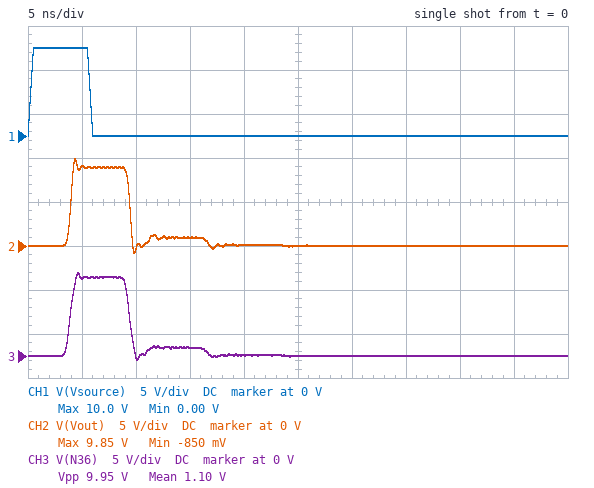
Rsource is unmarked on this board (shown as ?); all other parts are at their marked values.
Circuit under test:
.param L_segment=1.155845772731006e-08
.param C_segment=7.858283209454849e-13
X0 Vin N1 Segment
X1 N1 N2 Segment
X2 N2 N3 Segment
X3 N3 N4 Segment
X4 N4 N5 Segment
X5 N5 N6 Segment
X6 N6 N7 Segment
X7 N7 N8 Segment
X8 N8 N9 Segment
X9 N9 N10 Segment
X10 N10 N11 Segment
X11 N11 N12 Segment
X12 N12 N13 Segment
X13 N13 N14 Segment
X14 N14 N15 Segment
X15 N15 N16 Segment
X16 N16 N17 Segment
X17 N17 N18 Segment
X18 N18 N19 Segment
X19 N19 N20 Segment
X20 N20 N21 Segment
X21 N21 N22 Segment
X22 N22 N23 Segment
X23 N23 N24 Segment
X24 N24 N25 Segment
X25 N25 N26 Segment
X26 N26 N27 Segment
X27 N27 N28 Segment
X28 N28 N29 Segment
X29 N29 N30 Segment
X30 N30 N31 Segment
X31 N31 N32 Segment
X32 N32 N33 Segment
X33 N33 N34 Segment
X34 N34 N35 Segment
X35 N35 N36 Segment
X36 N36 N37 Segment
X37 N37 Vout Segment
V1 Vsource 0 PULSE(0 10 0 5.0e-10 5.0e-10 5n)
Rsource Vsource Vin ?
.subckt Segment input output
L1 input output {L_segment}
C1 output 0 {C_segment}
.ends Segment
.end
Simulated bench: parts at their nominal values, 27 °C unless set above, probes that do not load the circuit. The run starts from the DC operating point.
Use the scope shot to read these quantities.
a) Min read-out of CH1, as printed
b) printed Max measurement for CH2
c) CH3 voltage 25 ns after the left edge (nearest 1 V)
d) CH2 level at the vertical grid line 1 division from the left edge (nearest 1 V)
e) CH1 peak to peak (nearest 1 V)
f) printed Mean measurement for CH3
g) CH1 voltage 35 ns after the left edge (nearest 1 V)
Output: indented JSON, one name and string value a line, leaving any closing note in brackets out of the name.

{
  "Min read-out of CH1, as printed": "0.00 V",
  "printed Max measurement for CH2": "9.85 V",
  "CH3 voltage 25 ns after the left edge": "0 V",
  "CH2 level at the vertical grid line 1 division from the left edge": "9 V",
  "CH1 peak to peak": "10 V",
  "printed Mean measurement for CH3": "1.10 V",
  "CH1 voltage 35 ns after the left edge": "0 V"
}
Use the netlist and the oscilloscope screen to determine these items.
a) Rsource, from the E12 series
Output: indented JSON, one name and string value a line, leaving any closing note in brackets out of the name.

{
  "Rsource, from the E12 series": "150 Ω"
}
